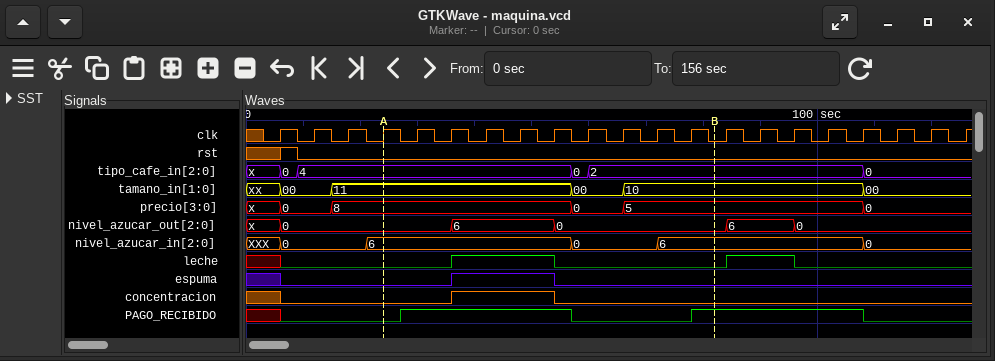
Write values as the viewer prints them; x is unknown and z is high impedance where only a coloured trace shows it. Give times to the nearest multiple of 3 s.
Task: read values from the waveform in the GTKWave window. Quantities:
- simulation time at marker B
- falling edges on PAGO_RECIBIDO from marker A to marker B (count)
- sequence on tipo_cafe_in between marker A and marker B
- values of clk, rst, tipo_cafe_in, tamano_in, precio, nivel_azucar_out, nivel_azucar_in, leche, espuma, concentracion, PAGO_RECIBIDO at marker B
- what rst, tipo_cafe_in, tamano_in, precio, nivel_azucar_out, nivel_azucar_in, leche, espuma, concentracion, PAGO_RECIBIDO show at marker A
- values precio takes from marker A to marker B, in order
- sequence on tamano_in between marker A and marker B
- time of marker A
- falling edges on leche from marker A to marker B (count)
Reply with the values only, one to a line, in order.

81 s
1
4, 0, 2
clk=0, rst=0, tipo_cafe_in=2, tamano_in=10, precio=5, nivel_azucar_out=0, nivel_azucar_in=6, leche=0, espuma=0, concentracion=0, PAGO_RECIBIDO=1
rst=0, tipo_cafe_in=4, tamano_in=11, precio=8, nivel_azucar_out=0, nivel_azucar_in=6, leche=0, espuma=0, concentracion=0, PAGO_RECIBIDO=0
8, 0, 5
11, 00, 10
24 s
1
